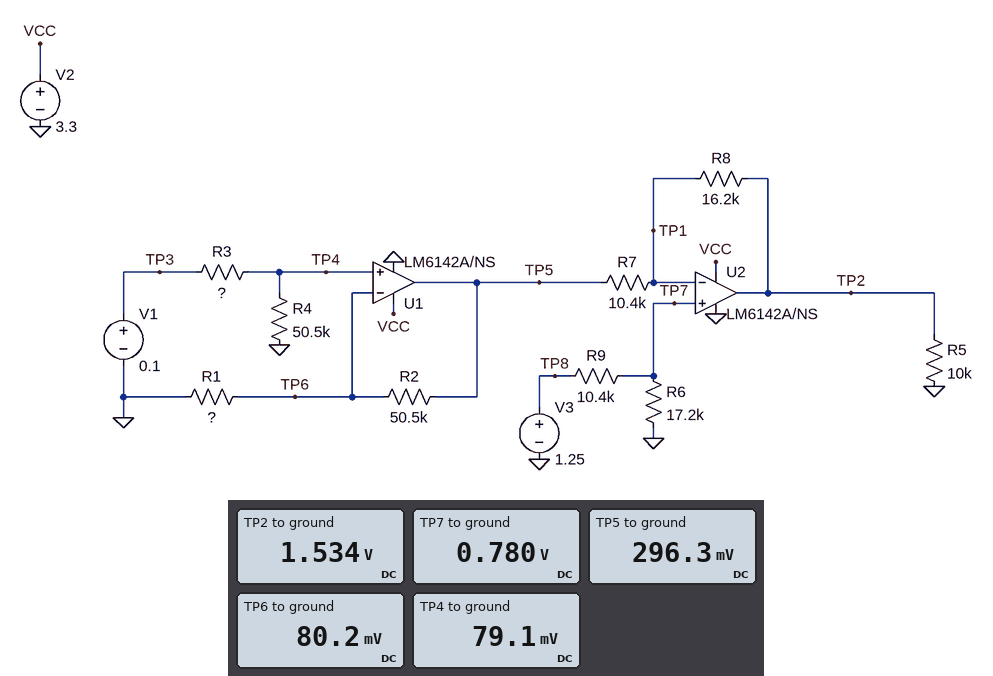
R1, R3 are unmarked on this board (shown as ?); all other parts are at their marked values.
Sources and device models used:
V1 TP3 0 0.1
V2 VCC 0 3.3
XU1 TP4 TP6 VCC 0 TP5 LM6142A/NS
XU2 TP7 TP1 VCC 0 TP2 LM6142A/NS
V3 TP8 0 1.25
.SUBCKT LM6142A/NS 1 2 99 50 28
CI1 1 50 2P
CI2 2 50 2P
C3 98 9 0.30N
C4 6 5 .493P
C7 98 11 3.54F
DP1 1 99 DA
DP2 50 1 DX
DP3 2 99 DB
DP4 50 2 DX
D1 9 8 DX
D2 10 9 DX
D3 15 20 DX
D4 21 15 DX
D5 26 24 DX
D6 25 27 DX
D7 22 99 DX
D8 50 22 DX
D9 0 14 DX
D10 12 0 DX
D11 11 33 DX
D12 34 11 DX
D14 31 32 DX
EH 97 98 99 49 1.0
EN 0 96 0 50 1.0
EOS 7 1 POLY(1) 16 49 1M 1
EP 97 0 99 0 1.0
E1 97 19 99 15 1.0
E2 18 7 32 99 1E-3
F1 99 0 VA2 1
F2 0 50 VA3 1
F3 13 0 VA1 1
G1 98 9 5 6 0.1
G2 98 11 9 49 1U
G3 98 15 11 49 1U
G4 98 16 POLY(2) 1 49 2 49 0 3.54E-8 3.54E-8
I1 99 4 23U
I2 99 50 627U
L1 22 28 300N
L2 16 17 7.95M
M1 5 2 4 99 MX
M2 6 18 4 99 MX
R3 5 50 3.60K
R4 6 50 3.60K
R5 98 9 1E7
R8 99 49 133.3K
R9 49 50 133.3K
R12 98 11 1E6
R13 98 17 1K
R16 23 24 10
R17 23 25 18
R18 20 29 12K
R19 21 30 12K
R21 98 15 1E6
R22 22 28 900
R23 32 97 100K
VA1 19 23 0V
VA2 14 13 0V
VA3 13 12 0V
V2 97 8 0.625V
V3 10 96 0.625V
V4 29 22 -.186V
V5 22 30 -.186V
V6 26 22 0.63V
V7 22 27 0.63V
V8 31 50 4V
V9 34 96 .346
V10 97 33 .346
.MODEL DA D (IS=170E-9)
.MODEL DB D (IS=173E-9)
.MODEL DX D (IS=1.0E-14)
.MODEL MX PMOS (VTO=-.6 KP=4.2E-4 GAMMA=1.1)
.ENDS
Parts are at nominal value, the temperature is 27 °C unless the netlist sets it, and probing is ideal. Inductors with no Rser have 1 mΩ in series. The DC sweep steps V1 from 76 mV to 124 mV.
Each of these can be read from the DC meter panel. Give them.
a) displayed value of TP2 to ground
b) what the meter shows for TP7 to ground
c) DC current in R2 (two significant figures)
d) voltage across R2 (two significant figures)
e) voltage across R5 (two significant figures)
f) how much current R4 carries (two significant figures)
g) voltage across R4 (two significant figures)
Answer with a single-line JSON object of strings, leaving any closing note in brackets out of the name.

{"displayed value of TP2 to ground": "1.534 V", "what the meter shows for TP7 to ground": "0.780 V", "DC current in R2": "4.3 µA", "voltage across R2": "220 mV", "voltage across R5": "1.5 V", "how much current R4 carries": "1.6 µA", "voltage across R4": "79 mV"}
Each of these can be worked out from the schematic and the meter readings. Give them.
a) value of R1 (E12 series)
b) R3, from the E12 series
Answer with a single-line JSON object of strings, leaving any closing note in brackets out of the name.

{"value of R1": "18 kΩ", "R3, from the E12 series": "15 kΩ"}
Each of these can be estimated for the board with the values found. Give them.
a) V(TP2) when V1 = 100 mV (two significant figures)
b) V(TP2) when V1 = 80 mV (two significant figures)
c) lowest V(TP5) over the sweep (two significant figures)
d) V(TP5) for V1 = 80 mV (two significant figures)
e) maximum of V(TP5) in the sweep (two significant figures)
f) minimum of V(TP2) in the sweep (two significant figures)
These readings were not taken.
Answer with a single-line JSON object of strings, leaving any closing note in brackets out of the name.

{"V(TP2) when V1 = 100 mV": "1.5 V", "V(TP2) when V1 = 80 mV": "1.6 V", "lowest V(TP5) over the sweep": "230 mV", "V(TP5) for V1 = 80 mV": "240 mV", "maximum of V(TP5) in the sweep": "370 mV", "minimum of V(TP2) in the sweep": "1.4 V"}
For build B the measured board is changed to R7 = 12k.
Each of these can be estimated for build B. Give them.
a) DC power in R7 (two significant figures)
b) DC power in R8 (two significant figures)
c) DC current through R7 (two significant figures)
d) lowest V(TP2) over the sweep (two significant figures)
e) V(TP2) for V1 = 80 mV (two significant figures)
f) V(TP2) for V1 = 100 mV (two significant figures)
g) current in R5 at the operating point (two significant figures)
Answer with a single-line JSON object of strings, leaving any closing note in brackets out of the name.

{"DC power in R7": "20 µW", "DC power in R8": "26 µW", "DC current through R7": "40 µA", "lowest V(TP2) over the sweep": "1.3 V", "V(TP2) for V1 = 80 mV": "1.5 V", "V(TP2) for V1 = 100 mV": "1.4 V", "current in R5 at the operating point": "140 µA"}
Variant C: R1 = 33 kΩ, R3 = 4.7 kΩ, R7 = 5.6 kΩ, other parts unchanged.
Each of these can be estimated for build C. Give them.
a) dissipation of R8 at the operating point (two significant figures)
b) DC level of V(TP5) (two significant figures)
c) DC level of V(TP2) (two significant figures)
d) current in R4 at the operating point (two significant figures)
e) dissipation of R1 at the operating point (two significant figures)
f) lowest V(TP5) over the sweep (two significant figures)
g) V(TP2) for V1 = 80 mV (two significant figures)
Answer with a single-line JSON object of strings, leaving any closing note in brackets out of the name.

{"dissipation of R8 at the operating point": "160 µW", "DC level of V(TP5)": "230 mV", "DC level of V(TP2)": "2.4 V", "current in R4 at the operating point": "1.8 µA", "dissipation of R1 at the operating point": "260 nW", "lowest V(TP5) over the sweep": "170 mV", "V(TP2) for V1 = 80 mV": "2.5 V"}
